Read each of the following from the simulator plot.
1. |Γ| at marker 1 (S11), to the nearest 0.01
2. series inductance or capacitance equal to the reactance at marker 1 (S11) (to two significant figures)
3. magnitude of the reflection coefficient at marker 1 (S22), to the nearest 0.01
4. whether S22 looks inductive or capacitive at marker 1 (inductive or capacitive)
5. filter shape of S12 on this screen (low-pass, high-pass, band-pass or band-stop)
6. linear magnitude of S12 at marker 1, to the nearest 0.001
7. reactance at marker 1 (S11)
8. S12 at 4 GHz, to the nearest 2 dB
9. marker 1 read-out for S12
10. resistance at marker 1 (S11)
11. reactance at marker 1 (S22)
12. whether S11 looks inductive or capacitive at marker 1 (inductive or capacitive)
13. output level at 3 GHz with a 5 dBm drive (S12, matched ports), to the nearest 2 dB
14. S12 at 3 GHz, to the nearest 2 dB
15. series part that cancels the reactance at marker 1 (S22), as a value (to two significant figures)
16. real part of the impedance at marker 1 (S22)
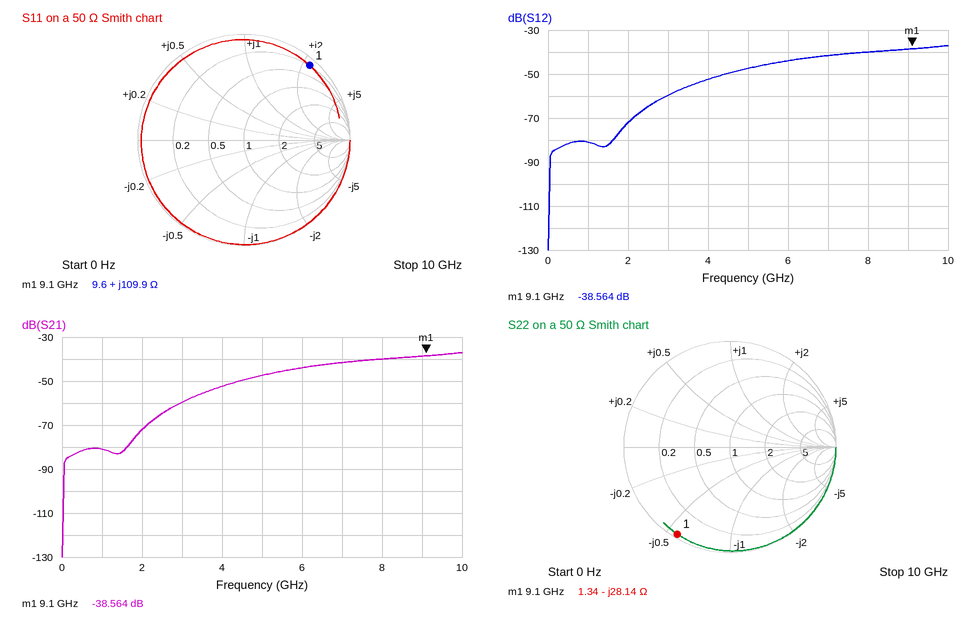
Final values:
0.94
1.9 nH
0.96
capacitive
high-pass
0.012
+109.9 Ω
-52 dB
-38.564 dB
9.6 Ω
-28.14 Ω
inductive
-54 dBm
-60 dB
490 pH
1.34 Ω
